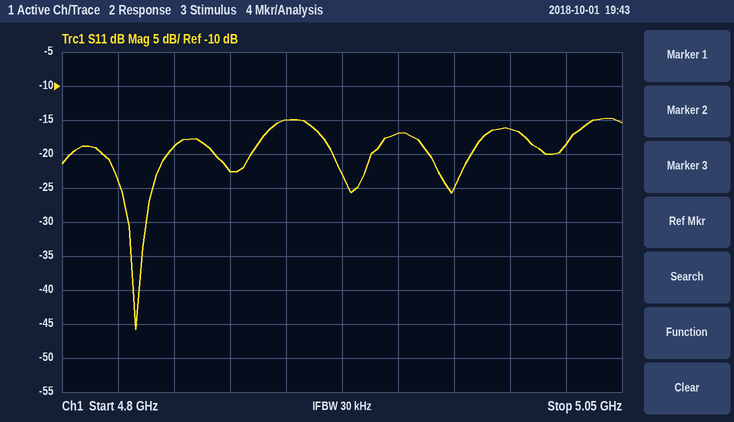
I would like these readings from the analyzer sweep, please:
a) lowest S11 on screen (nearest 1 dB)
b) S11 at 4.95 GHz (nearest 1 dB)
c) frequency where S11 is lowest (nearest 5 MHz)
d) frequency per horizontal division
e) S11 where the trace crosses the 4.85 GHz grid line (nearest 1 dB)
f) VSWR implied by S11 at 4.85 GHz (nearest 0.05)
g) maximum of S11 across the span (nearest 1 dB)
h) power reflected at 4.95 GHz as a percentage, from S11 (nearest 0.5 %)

-46 dB
-17 dB
4.835 GHz
25 MHz
-19 dB
1.25
-15 dB
2.0 %
